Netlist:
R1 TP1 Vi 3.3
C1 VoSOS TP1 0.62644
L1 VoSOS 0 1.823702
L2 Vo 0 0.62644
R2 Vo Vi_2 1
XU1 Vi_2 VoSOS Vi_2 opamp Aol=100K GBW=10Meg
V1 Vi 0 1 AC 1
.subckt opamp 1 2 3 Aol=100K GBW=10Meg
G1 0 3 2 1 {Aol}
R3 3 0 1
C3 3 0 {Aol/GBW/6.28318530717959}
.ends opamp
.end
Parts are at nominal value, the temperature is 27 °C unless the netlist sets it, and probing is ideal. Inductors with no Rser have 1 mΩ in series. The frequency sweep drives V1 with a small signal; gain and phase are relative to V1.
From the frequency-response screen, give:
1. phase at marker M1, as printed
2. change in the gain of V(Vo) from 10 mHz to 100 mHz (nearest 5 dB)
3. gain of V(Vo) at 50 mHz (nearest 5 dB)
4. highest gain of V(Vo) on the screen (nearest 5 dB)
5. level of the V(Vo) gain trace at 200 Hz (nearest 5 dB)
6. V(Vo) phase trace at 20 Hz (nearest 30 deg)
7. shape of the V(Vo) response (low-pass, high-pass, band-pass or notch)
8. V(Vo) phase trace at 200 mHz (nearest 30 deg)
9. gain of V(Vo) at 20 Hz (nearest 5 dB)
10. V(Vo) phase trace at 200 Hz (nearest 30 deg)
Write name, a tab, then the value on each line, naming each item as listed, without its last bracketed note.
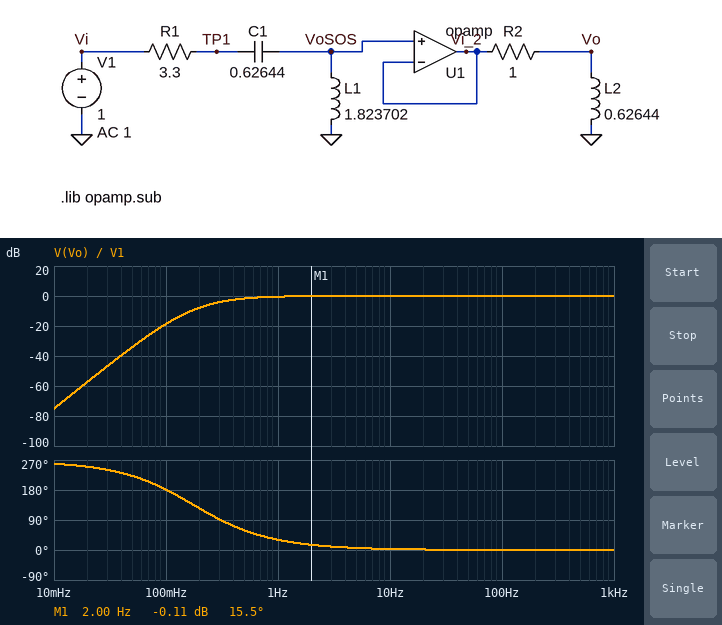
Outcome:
phase at marker M1, as printed	15.5 deg
change in the gain of V(Vo) from 10 mHz to 100 mHz	55 dB
gain of V(Vo) at 50 mHz	-35 dB
highest gain of V(Vo) on the screen	0 dB
level of the V(Vo) gain trace at 200 Hz	0 dB
V(Vo) phase trace at 20 Hz	0 deg
shape of the V(Vo) response	high-pass
V(Vo) phase trace at 200 mHz	120 deg
gain of V(Vo) at 20 Hz	0 dB
V(Vo) phase trace at 200 Hz	0 deg
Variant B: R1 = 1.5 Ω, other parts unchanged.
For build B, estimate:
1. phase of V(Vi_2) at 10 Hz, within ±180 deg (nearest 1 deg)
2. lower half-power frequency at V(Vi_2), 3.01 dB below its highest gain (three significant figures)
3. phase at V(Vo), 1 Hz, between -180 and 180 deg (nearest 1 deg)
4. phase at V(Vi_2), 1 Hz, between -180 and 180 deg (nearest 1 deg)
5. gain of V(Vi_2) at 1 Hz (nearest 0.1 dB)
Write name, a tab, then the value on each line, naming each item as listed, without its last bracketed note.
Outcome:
phase of V(Vi_2) at 10 Hz, within ±180 deg	1 deg
lower half-power frequency at V(Vi_2), 3.01 dB below its highest gain	126 mHz
phase at V(Vo), 1 Hz, between -180 and 180 deg	22 deg
phase at V(Vi_2), 1 Hz, between -180 and 180 deg	8 deg
gain of V(Vi_2) at 1 Hz	0.1 dB
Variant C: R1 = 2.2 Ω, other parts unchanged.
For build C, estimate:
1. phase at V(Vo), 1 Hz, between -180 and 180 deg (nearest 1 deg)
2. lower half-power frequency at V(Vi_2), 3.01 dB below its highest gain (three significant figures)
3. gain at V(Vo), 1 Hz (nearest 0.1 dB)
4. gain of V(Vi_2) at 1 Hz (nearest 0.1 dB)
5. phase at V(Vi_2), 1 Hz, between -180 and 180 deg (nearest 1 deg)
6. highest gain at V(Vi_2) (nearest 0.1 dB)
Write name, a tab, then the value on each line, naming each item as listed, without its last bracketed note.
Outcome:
phase at V(Vo), 1 Hz, between -180 and 180 deg	25 deg
lower half-power frequency at V(Vi_2), 3.01 dB below its highest gain	139 mHz
gain at V(Vo), 1 Hz	-0.2 dB
gain of V(Vi_2) at 1 Hz	0 dB
phase at V(Vi_2), 1 Hz, between -180 and 180 deg	11 deg
highest gain at V(Vi_2)	0.1 dB
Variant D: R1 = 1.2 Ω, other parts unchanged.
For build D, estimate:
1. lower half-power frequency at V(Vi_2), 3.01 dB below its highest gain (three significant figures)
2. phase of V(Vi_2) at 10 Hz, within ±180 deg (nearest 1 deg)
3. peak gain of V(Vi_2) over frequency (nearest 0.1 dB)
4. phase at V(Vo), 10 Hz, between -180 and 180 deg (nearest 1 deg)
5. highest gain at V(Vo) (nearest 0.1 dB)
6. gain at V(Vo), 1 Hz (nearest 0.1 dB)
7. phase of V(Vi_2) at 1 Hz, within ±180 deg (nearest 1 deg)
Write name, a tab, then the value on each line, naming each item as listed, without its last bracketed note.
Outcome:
lower half-power frequency at V(Vi_2), 3.01 dB below its highest gain	125 mHz
phase of V(Vi_2) at 10 Hz, within ±180 deg	1 deg
peak gain of V(Vi_2) over frequency	3.6 dB
phase at V(Vo), 10 Hz, between -180 and 180 deg	2 deg
highest gain at V(Vo)	0 dB
gain at V(Vo), 1 Hz	-0.1 dB
phase of V(Vi_2) at 1 Hz, within ±180 deg	6 deg
